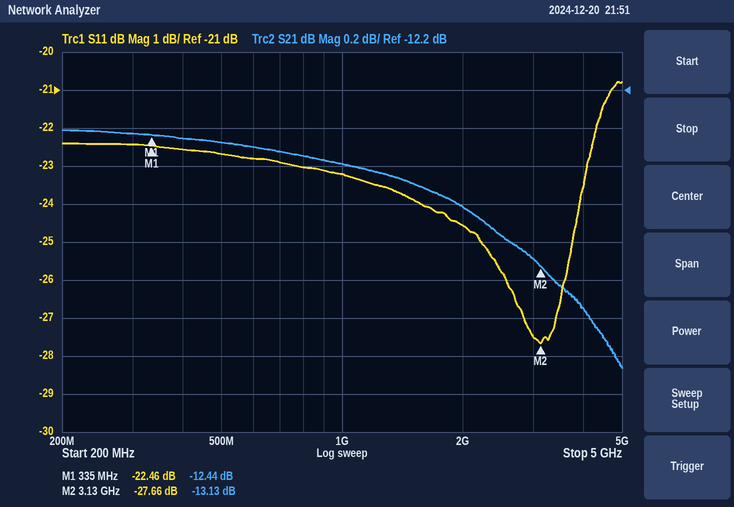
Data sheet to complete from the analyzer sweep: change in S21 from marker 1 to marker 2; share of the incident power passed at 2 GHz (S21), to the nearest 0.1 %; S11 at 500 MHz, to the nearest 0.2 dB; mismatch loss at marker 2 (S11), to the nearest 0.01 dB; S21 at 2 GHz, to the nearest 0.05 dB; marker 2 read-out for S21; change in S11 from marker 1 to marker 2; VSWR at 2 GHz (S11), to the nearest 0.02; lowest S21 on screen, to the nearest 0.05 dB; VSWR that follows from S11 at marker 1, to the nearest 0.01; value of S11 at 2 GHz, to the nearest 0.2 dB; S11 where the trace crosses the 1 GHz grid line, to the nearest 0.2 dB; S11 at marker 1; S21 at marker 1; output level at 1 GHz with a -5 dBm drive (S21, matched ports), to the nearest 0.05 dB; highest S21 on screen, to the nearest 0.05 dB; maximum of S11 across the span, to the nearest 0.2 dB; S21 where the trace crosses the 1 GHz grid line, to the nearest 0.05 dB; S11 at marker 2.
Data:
-0.69 dB
5.2 %
-22.6 dB
0.01 dB
-12.80 dB
-13.13 dB
-5.20 dB
1.12
-13.65 dB
1.16
-24.6 dB
-23.2 dB
-22.46 dB
-12.44 dB
-17.60 dBm
-12.40 dB
-20.8 dB
-12.60 dB
-27.66 dB
